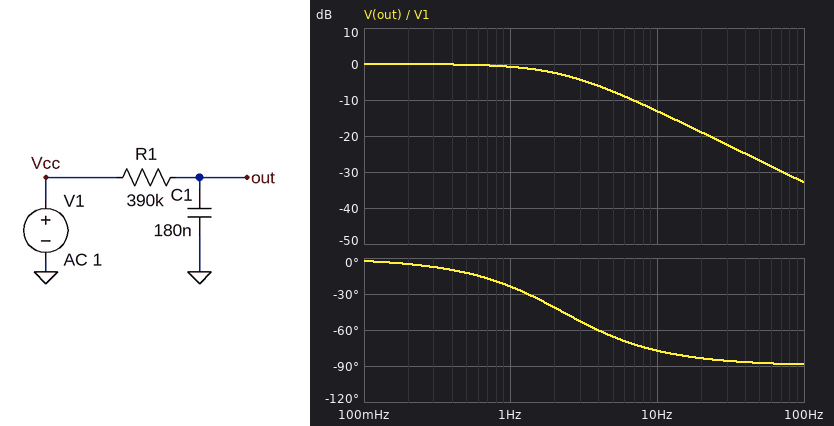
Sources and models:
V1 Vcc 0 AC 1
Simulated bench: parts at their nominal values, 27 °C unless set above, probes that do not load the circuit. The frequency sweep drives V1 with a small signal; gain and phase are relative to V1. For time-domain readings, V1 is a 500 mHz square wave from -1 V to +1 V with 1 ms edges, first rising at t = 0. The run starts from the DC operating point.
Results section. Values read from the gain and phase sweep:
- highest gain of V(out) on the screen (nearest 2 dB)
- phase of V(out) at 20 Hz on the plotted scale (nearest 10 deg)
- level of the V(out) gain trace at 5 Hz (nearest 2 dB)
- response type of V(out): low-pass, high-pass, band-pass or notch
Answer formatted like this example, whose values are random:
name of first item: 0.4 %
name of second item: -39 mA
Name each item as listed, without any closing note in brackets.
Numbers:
highest gain of V(out) on the screen: 0 dB
phase of V(out) at 20 Hz on the plotted scale: -80 deg
level of the V(out) gain trace at 5 Hz: -8 dB
response type of V(out): low-pass, high-pass, band-pass or notch: low-pass
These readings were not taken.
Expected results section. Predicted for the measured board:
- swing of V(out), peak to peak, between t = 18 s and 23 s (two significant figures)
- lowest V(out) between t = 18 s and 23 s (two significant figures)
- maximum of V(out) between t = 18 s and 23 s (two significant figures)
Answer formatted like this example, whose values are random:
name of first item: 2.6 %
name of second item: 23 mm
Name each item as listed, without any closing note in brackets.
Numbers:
swing of V(out), peak to peak, between t = 18 s and 23 s: 2.0 V
lowest V(out) between t = 18 s and 23 s: -1.0 V
maximum of V(out) between t = 18 s and 23 s: 1.0 V
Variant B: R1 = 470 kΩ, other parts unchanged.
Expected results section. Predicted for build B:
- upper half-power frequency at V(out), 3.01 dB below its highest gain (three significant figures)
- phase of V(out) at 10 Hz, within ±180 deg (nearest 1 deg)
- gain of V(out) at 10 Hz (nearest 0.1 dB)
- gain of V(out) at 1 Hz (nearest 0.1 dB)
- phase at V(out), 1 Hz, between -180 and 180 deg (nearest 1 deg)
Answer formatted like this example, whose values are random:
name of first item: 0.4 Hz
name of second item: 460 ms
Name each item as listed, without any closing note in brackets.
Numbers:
upper half-power frequency at V(out), 3.01 dB below its highest gain: 1.88 Hz
phase of V(out) at 10 Hz, within ±180 deg: -79 deg
gain of V(out) at 10 Hz: -14.7 dB
gain of V(out) at 1 Hz: -1.1 dB
phase at V(out), 1 Hz, between -180 and 180 deg: -28 deg
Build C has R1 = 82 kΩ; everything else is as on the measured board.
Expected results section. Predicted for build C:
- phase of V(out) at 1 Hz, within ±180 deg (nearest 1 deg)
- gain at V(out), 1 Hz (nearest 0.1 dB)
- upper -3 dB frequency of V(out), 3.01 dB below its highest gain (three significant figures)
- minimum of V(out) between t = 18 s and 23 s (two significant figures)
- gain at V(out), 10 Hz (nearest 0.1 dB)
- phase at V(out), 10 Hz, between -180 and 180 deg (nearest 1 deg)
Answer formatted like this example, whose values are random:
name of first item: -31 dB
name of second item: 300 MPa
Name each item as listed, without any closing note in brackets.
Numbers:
phase of V(out) at 1 Hz, within ±180 deg: -5 deg
gain at V(out), 1 Hz: 0 dB
upper -3 dB frequency of V(out), 3.01 dB below its highest gain: 10.8 Hz
minimum of V(out) between t = 18 s and 23 s: -1.0 V
gain at V(out), 10 Hz: -2.7 dB
phase at V(out), 10 Hz, between -180 and 180 deg: -43 deg
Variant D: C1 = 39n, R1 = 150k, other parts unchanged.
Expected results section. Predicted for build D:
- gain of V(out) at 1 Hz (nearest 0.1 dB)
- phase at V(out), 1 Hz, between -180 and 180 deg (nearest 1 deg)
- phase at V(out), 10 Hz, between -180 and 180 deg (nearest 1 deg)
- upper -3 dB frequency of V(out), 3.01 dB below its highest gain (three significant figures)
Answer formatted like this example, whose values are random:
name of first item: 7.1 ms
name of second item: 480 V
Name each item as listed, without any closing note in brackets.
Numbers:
gain of V(out) at 1 Hz: 0 dB
phase at V(out), 1 Hz, between -180 and 180 deg: -2 deg
phase at V(out), 10 Hz, between -180 and 180 deg: -20 deg
upper -3 dB frequency of V(out), 3.01 dB below its highest gain: 27.2 Hz
